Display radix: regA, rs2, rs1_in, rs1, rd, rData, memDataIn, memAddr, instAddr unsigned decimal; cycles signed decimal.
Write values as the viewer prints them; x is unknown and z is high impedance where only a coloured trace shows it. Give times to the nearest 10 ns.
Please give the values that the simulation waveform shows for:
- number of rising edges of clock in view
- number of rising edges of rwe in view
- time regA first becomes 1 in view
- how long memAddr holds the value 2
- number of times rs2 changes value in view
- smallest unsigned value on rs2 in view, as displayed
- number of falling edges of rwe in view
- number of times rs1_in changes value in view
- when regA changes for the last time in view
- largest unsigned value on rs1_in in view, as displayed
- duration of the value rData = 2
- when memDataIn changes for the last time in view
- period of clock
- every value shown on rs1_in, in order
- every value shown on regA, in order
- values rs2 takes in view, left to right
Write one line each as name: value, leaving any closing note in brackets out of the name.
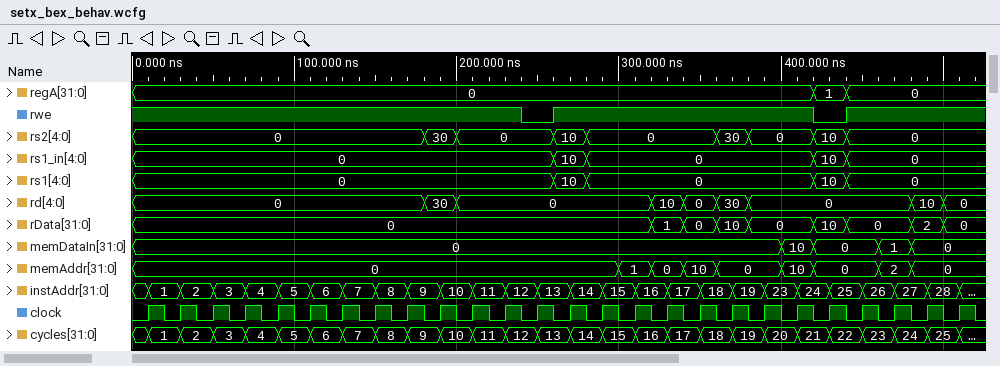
number of rising edges of clock in view: 26
number of rising edges of rwe in view: 2
time regA first becomes 1 in view: 420 ns
how long memAddr holds the value 2: 20 ns
number of times rs2 changes value in view: 8
smallest unsigned value on rs2 in view, as displayed: 0
number of falling edges of rwe in view: 2
number of times rs1_in changes value in view: 4
when regA changes for the last time in view: 440 ns
largest unsigned value on rs1_in in view, as displayed: 10
duration of the value rData = 2: 20 ns
when memDataIn changes for the last time in view: 480 ns
period of clock: 20 ns
every value shown on rs1_in, in order: 0, 10, 0, 10, 0
every value shown on regA, in order: 0, 1, 0
values rs2 takes in view, left to right: 0, 30, 0, 10, 0, 30, 0, 10, 0
